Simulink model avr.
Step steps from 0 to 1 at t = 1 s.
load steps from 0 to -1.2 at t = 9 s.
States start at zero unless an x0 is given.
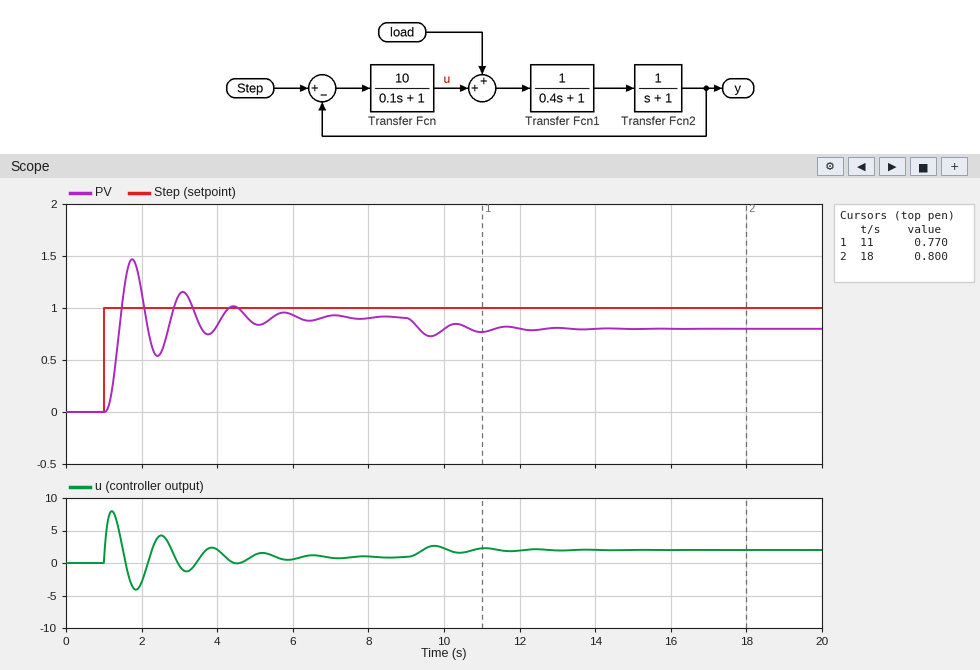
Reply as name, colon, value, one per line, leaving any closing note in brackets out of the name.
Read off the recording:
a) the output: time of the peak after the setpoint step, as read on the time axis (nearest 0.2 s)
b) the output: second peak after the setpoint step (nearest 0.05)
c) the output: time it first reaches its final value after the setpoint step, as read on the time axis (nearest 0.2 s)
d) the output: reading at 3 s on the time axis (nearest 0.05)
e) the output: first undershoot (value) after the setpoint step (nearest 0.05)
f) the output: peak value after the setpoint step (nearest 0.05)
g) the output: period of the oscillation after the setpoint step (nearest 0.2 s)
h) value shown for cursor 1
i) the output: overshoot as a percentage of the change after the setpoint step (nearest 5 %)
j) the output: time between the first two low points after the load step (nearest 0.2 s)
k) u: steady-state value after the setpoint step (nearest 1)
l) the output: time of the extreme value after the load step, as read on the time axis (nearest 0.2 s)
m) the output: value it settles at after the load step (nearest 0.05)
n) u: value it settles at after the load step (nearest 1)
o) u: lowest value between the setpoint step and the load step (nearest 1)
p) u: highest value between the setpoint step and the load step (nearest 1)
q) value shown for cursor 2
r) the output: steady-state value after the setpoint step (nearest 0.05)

the output: time of the peak after the setpoint step, as read on the time axis: 1.8 s
the output: second peak after the setpoint step: 1.15
the output: time it first reaches its final value after the setpoint step, as read on the time axis: 1.4 s
the output: reading at 3 s on the time axis: 1.15
the output: first undershoot (value) after the setpoint step: 0.55
the output: peak value after the setpoint step: 1.45
the output: period of the oscillation after the setpoint step: 1.4 s
value shown for cursor 1: 0.770
the output: overshoot as a percentage of the change after the setpoint step: 60 %
the output: time between the first two low points after the load step: 1.4 s
u: steady-state value after the setpoint step: 1
the output: time of the extreme value after the load step, as read on the time axis: 9.6 s
the output: value it settles at after the load step: 0.80
u: value it settles at after the load step: 2
u: lowest value between the setpoint step and the load step: -4
u: highest value between the setpoint step and the load step: 8
value shown for cursor 2: 0.800
the output: steady-state value after the setpoint step: 0.90
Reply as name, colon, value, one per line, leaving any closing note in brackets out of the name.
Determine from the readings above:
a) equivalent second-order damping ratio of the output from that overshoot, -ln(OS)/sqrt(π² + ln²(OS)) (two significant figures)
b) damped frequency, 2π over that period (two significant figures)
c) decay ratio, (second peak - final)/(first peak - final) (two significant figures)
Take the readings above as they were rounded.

equivalent second-order damping ratio of the output from that overshoot, -ln(OS)/sqrt(π² + ln²(OS)): 0.16
damped frequency, 2π over that period: 4.5 rad/s
decay ratio, (second peak - final)/(first peak - final): 0.45
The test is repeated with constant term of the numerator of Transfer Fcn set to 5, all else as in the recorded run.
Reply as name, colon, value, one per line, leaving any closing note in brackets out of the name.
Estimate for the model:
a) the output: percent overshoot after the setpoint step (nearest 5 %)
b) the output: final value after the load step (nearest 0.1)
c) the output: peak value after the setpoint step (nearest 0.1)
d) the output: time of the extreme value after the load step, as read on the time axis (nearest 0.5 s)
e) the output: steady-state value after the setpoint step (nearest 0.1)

the output: percent overshoot after the setpoint step: 35 %
the output: final value after the load step: 0.6
the output: peak value after the setpoint step: 1.1
the output: time of the extreme value after the load step, as read on the time axis: 10.0 s
the output: steady-state value after the setpoint step: 0.8
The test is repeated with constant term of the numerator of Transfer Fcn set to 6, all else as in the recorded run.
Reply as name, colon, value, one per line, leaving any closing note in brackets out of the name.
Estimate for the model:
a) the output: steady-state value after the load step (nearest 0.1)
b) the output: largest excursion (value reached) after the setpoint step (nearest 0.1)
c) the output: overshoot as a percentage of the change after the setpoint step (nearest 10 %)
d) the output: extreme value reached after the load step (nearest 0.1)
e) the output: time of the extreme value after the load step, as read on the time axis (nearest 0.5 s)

the output: steady-state value after the load step: 0.7
the output: largest excursion (value reached) after the setpoint step: 1.2
the output: overshoot as a percentage of the change after the setpoint step: 40 %
the output: extreme value reached after the load step: 0.6
the output: time of the extreme value after the load step, as read on the time axis: 10.0 s
